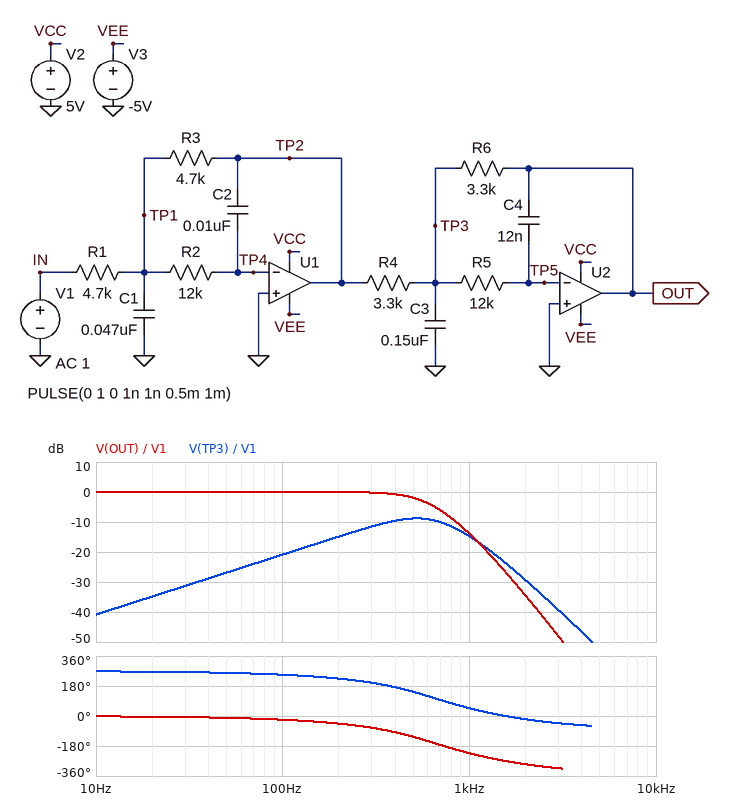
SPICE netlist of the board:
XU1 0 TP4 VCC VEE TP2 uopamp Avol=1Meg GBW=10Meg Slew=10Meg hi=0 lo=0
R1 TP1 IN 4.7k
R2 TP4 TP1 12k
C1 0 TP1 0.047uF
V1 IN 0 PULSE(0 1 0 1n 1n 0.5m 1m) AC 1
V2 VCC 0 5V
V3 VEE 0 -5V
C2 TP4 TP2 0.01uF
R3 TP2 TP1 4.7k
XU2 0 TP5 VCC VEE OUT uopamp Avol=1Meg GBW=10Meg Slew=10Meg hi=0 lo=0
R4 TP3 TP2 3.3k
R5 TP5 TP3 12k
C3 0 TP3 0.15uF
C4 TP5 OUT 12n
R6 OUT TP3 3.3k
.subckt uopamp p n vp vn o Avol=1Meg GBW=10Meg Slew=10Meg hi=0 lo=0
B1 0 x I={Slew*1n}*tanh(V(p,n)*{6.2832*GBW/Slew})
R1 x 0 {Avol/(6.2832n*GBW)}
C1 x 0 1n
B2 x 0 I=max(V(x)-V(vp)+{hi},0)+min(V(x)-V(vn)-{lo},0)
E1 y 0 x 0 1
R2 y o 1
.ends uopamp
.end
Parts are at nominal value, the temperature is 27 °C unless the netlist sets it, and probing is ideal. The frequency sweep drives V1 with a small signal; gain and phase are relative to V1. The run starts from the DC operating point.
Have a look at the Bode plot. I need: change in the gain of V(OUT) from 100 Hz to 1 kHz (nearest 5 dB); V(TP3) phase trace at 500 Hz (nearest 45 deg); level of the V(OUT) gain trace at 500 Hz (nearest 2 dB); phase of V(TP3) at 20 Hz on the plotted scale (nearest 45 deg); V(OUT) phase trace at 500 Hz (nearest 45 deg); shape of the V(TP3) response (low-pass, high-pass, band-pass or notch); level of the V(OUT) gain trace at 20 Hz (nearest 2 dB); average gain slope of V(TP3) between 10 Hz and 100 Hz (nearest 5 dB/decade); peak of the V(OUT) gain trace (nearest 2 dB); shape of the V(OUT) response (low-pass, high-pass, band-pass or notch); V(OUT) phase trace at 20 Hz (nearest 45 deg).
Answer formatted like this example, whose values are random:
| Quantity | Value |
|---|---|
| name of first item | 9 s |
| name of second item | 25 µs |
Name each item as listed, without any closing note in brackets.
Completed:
| Quantity | Value |
|---|---|
| change in the gain of V(OUT) from 100 Hz to 1 kHz | -15 dB |
| V(TP3) phase trace at 500 Hz | 135 deg |
| level of the V(OUT) gain trace at 500 Hz | -2 dB |
| phase of V(TP3) at 20 Hz on the plotted scale | 270 deg |
| V(OUT) phase trace at 500 Hz | -135 deg |
| shape of the V(TP3) response | band-pass |
| level of the V(OUT) gain trace at 20 Hz | 0 dB |
| average gain slope of V(TP3) between 10 Hz and 100 Hz | 20 dB/decade |
| peak of the V(OUT) gain trace | 0 dB |
| shape of the V(OUT) response | low-pass |
| V(OUT) phase trace at 20 Hz | 0 deg |
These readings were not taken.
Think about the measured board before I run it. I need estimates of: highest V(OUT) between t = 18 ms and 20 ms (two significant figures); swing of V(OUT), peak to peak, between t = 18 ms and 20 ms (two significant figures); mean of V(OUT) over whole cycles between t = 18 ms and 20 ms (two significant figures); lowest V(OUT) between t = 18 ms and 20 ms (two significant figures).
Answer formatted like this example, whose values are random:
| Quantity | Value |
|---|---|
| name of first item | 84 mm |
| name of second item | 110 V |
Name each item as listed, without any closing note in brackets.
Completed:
| Quantity | Value |
|---|---|
| highest V(OUT) between t = 18 ms and 20 ms | 630 mV |
| swing of V(OUT), peak to peak, between t = 18 ms and 20 ms | 260 mV |
| mean of V(OUT) over whole cycles between t = 18 ms and 20 ms | 500 mV |
| lowest V(OUT) between t = 18 ms and 20 ms | 370 mV |
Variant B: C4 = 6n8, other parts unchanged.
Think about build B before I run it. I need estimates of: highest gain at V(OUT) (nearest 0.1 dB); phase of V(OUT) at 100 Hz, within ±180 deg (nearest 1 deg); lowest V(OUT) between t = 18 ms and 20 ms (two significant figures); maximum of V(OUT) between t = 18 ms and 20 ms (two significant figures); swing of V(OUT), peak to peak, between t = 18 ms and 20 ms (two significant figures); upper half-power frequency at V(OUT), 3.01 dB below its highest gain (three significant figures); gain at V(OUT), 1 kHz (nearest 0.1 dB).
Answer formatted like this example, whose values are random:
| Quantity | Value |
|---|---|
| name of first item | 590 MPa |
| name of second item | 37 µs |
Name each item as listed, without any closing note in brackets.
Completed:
| Quantity | Value |
|---|---|
| highest gain at V(OUT) | 0.3 dB |
| phase of V(OUT) at 100 Hz, within ±180 deg | -17 deg |
| lowest V(OUT) between t = 18 ms and 20 ms | 230 mV |
| maximum of V(OUT) between t = 18 ms and 20 ms | 770 mV |
| swing of V(OUT), peak to peak, between t = 18 ms and 20 ms | 540 mV |
| upper half-power frequency at V(OUT), 3.01 dB below its highest gain | 796 Hz |
| gain at V(OUT), 1 kHz | -7.5 dB |
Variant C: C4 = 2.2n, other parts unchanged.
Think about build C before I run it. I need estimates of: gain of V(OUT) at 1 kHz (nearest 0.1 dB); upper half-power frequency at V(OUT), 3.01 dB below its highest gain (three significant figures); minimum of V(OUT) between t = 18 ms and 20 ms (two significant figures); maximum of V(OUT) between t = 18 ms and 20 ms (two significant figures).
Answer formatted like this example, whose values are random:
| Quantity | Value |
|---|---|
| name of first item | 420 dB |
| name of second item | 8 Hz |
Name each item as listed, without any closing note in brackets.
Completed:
| Quantity | Value |
|---|---|
| gain of V(OUT) at 1 kHz | -0.9 dB |
| upper half-power frequency at V(OUT), 3.01 dB below its highest gain | 1.39 kHz |
| minimum of V(OUT) between t = 18 ms and 20 ms | -75 mV |
| maximum of V(OUT) between t = 18 ms and 20 ms | 1.1 V |
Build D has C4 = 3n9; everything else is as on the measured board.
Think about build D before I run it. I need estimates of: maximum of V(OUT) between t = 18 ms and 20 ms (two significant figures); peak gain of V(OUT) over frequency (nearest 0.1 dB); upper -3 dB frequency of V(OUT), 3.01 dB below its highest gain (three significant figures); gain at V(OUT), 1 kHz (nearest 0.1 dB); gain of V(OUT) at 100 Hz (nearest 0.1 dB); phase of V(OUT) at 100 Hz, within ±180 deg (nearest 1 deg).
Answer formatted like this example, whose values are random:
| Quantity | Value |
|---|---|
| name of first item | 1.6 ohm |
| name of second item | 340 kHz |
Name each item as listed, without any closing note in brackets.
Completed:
| Quantity | Value |
|---|---|
| maximum of V(OUT) between t = 18 ms and 20 ms | 1.0 V |
| peak gain of V(OUT) over frequency | 0.2 dB |
| upper -3 dB frequency of V(OUT), 3.01 dB below its highest gain | 1.07 kHz |
| gain at V(OUT), 1 kHz | -1.7 dB |
| gain of V(OUT) at 100 Hz | 0 dB |
| phase of V(OUT) at 100 Hz, within ±180 deg | -14 deg |
